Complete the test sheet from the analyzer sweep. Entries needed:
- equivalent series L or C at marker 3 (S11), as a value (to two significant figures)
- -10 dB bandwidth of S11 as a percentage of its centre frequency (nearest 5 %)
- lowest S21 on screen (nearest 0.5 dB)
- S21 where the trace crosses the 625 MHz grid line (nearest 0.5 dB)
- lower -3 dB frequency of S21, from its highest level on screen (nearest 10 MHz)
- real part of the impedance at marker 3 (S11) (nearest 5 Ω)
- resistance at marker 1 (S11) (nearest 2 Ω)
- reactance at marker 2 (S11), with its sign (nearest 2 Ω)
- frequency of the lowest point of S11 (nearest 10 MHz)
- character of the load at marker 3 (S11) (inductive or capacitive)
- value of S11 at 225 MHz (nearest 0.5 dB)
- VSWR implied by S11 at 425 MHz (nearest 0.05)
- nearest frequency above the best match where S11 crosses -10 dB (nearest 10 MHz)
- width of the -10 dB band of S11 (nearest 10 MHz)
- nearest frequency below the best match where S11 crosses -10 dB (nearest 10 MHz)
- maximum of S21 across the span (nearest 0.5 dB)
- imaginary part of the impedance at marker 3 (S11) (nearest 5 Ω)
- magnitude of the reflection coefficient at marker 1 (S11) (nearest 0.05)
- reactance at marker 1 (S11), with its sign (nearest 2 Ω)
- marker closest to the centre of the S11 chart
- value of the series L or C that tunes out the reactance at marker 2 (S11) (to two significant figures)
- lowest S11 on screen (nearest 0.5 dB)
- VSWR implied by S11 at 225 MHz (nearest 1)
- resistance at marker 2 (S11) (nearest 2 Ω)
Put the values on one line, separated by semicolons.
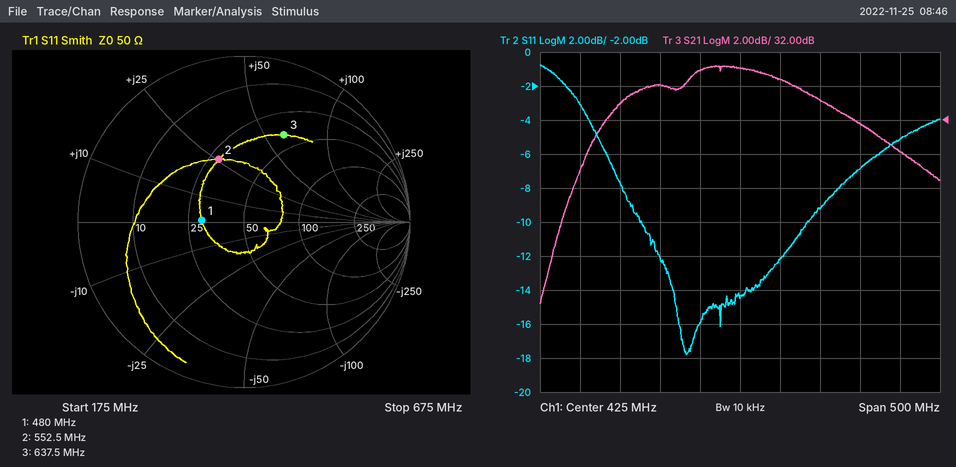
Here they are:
15 nH; 50 %; 21.0 dB; 30.0 dB; 260 MHz; 40 Ω; 30 Ω; +26 Ω; 360 MHz; inductive; -3.0 dB; 1.45; 510 MHz; 210 MHz; 300 MHz; 35.0 dB; +60 Ω; 0.25; 0 Ω; marker 1; 11 pF; -18.0 dB; 6; 28 Ω
